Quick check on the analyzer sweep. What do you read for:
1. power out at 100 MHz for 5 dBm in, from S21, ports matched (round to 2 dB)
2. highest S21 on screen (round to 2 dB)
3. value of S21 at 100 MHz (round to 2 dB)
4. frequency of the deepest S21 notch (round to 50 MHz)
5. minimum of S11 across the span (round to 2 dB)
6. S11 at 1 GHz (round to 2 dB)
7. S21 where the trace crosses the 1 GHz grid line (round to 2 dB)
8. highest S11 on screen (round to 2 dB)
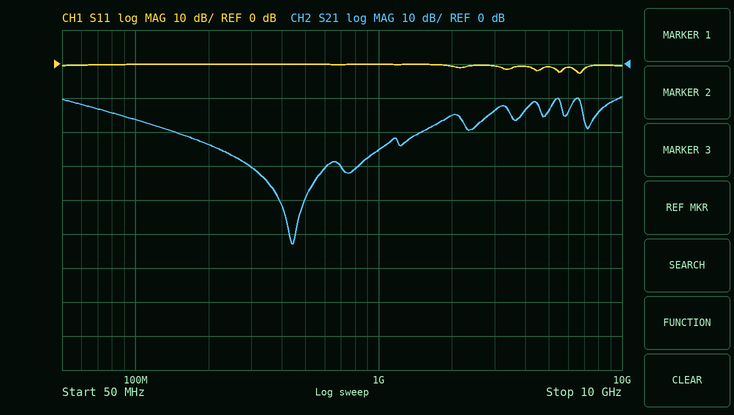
-12 dBm
-10 dB
-16 dB
450 MHz
-2 dB
0 dB
-26 dB
0 dB
